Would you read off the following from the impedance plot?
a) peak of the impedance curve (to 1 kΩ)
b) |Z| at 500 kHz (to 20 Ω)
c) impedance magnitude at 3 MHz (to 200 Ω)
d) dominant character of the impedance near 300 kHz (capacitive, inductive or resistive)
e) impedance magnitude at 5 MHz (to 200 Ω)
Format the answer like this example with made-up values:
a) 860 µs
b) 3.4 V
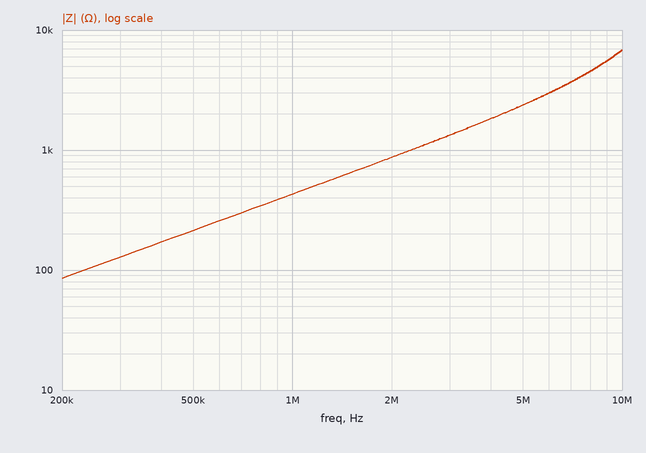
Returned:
a) 7 kΩ
b) 220 Ω
c) 1.4 kΩ
d) inductive
e) 2.4 kΩ
